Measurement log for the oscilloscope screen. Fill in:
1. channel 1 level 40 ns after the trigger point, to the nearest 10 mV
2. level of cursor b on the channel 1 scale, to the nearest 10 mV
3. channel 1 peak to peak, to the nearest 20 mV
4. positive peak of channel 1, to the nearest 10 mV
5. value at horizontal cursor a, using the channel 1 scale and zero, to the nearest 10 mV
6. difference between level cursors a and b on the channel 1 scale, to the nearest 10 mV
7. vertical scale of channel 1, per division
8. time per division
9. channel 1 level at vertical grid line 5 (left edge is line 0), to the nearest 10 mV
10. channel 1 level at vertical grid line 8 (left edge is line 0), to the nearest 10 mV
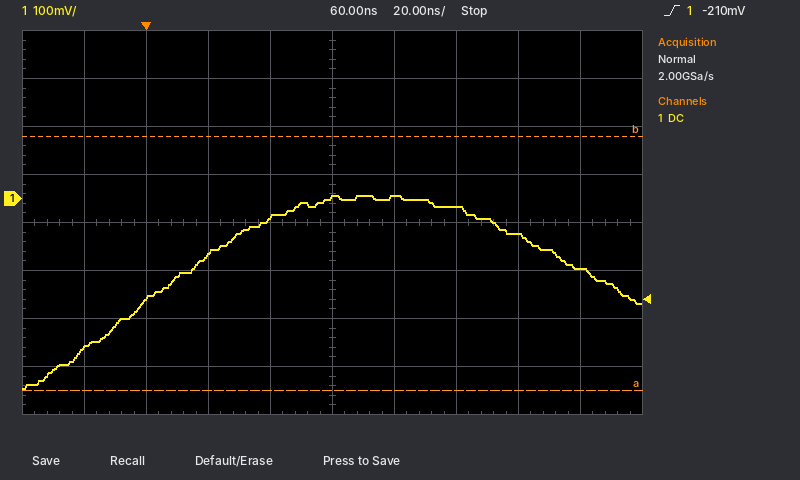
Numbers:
-40 mV
130 mV
400 mV
10 mV
-400 mV
530 mV
100 mV
20 ns
0 mV
-70 mV
